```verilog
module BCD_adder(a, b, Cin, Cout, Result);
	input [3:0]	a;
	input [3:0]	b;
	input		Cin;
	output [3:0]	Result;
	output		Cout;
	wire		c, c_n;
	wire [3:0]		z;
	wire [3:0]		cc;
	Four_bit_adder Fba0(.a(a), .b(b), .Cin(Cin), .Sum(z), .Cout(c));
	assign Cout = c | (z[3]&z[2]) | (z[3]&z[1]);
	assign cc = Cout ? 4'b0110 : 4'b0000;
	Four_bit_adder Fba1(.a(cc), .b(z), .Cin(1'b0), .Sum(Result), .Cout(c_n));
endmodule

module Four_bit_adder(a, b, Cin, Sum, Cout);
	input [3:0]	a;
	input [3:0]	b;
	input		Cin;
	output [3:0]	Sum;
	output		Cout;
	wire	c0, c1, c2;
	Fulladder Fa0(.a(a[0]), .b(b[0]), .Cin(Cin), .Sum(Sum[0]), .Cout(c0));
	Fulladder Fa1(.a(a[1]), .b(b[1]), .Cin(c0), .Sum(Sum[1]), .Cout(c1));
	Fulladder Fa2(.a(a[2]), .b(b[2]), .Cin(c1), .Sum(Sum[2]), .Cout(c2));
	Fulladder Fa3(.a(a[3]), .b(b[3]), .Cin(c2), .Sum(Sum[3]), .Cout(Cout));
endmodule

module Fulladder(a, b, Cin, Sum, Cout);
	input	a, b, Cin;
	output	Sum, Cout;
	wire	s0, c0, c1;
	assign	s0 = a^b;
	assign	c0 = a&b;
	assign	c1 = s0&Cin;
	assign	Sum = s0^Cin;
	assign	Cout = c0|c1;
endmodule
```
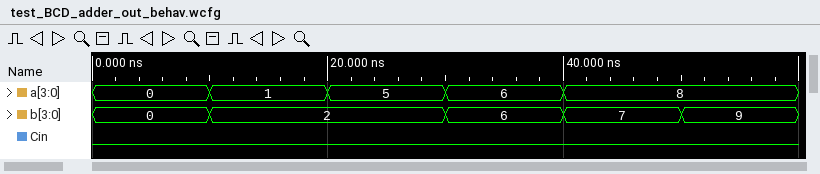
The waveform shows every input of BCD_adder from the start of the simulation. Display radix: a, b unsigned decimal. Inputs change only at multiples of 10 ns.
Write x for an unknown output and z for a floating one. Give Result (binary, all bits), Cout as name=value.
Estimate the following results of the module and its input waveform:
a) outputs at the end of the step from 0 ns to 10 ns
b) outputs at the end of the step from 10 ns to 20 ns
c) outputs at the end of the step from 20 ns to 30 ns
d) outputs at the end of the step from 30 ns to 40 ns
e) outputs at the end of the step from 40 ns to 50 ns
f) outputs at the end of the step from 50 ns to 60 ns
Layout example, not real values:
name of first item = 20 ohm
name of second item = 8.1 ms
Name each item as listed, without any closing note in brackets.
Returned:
outputs at the end of the step from 0 ns to 10 ns = Result=0000, Cout=0
outputs at the end of the step from 10 ns to 20 ns = Result=0011, Cout=0
outputs at the end of the step from 20 ns to 30 ns = Result=0111, Cout=0
outputs at the end of the step from 30 ns to 40 ns = Result=0010, Cout=1
outputs at the end of the step from 40 ns to 50 ns = Result=0101, Cout=1
outputs at the end of the step from 50 ns to 60 ns = Result=0111, Cout=1
